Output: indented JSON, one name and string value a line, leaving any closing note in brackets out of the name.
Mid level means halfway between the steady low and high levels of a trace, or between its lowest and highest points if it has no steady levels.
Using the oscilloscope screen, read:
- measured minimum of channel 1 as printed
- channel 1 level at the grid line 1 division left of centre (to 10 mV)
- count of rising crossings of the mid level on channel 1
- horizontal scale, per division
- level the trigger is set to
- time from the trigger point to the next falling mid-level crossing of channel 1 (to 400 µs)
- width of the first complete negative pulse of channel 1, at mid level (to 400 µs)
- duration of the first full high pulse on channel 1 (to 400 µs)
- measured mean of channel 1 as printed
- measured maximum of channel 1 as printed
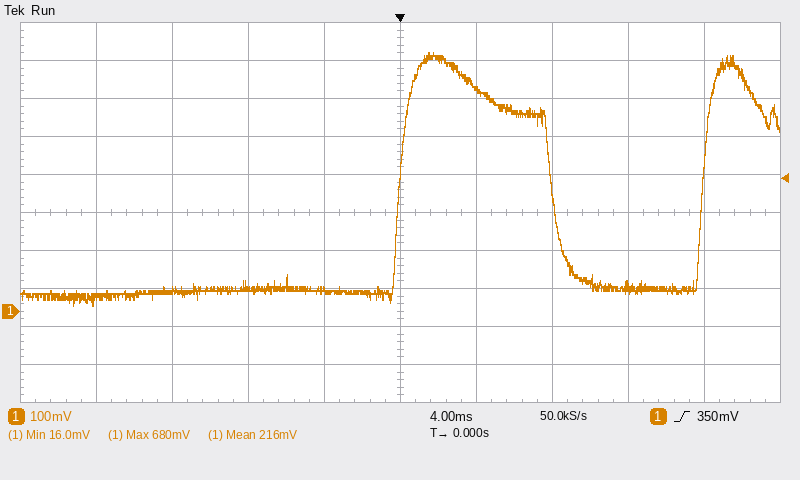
{
  "measured minimum of channel 1 as printed": "16.0 mV",
  "channel 1 level at the grid line 1 division left of centre": "60 mV",
  "count of rising crossings of the mid level on channel 1": "2",
  "horizontal scale, per division": "4 ms",
  "level the trigger is set to": "350 mV",
  "time from the trigger point to the next falling mid-level crossing of channel 1": "8.0 ms",
  "width of the first complete negative pulse of channel 1, at mid level": "8.0 ms",
  "duration of the first full high pulse on channel 1": "8.0 ms",
  "measured mean of channel 1 as printed": "216 mV",
  "measured maximum of channel 1 as printed": "680 mV"
}
